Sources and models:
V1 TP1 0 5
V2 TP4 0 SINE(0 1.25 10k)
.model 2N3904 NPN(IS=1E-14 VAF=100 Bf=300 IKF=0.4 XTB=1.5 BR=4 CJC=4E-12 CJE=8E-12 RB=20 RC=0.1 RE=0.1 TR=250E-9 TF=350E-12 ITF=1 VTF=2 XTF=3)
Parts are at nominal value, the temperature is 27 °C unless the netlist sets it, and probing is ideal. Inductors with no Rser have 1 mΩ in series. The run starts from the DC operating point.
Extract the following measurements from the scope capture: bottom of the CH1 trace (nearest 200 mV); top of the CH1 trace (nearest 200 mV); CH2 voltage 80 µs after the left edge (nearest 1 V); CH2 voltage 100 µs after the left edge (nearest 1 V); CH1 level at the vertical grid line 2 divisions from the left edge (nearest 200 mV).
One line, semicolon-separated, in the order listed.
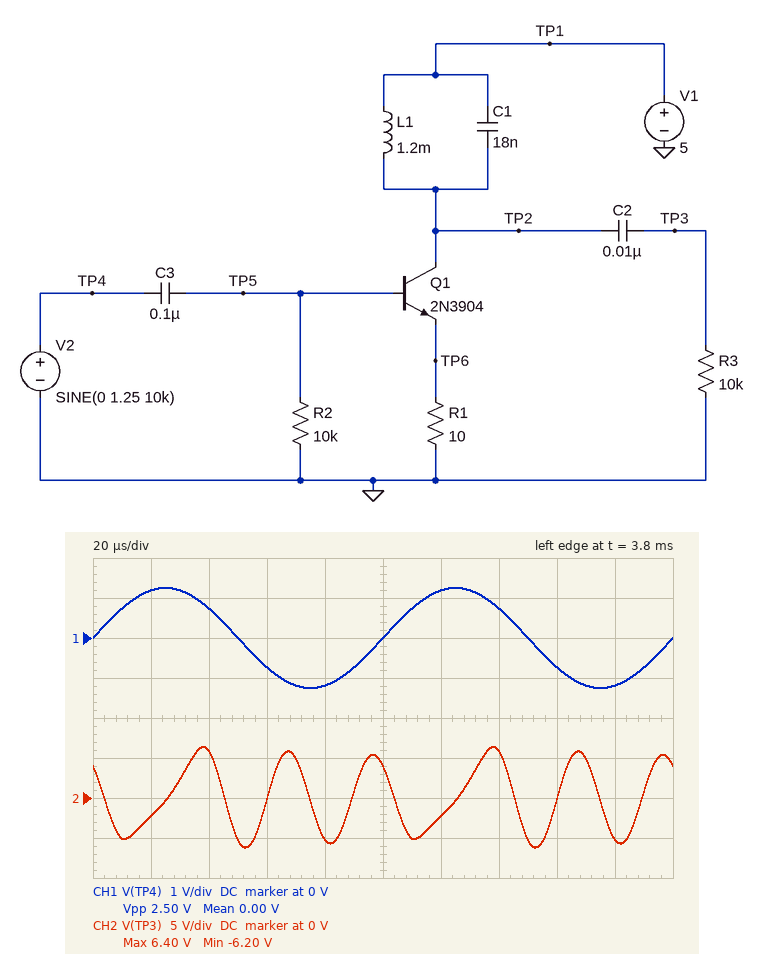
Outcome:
-1.2 V; 1.2 V; -5 V; 4 V; 800 mV
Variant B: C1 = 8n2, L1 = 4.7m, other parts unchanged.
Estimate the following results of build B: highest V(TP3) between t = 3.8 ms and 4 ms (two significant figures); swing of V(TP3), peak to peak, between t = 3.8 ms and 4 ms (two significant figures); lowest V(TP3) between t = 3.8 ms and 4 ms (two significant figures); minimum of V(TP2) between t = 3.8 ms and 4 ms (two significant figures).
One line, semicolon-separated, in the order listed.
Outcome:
8.8 V; 16 V; -7.2 V; -2.0 V
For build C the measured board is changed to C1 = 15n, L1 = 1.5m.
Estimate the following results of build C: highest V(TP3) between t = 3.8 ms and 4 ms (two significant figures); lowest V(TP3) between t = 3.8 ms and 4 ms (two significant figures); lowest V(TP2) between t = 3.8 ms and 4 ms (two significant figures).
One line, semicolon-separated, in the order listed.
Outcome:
7.1 V; -6.3 V; -1.2 V
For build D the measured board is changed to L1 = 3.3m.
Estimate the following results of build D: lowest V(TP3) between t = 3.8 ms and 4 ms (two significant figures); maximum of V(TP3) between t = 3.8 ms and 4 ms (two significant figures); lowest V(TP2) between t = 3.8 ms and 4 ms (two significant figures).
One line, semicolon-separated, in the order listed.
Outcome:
-6.5 V; 6.9 V; -1.5 V
